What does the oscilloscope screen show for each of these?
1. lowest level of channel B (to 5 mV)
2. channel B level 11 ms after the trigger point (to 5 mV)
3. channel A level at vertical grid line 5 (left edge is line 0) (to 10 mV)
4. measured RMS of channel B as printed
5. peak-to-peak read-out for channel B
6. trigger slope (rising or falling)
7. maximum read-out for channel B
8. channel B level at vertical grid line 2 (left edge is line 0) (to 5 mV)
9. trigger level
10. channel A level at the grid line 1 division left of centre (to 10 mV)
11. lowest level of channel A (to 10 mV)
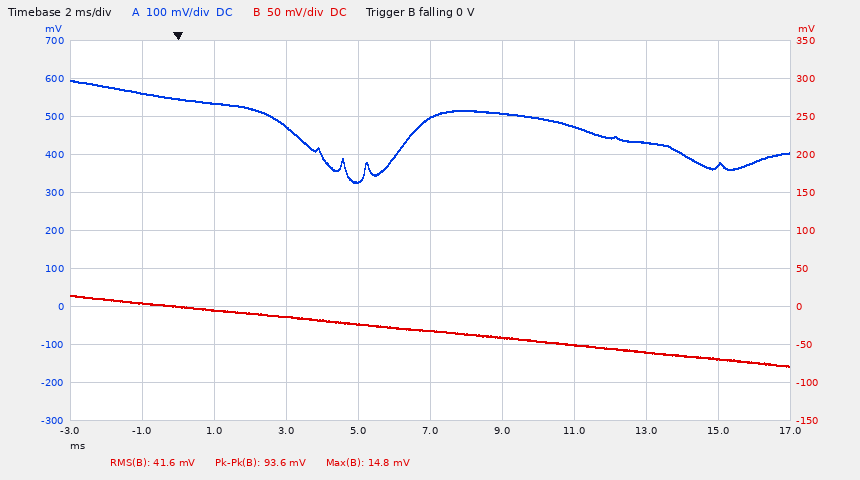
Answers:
-80 mV
-50 mV
500 mV
41.6 mV
93.6 mV
falling
14.8 mV
-5 mV
0 V
330 mV
330 mV
